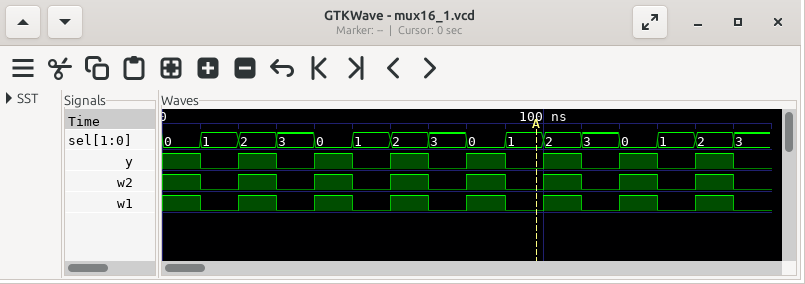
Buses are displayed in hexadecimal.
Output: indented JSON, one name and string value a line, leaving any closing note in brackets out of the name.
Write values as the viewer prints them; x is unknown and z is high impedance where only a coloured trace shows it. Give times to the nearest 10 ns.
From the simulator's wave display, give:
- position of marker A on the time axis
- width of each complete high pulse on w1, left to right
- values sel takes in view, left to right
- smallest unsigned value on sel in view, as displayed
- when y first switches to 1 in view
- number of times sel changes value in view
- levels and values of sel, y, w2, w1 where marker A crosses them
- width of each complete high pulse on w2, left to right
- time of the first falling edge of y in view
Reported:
{
  "position of marker A on the time axis": "100 ns",
  "width of each complete high pulse on w1, left to right": "10 ns, 10 ns, 10 ns, 10 ns, 10 ns, 10 ns, 10 ns",
  "values sel takes in view, left to right": "0, 1, 2, 3, 0, 1, 2, 3, 0, 1, 2, 3, 0, 1, 2, 3",
  "smallest unsigned value on sel in view, as displayed": "0",
  "when y first switches to 1 in view": "20 ns",
  "number of times sel changes value in view": "15",
  "levels and values of sel, y, w2, w1 where marker A crosses them": "sel=1, y=0, w2=0, w1=0",
  "width of each complete high pulse on w2, left to right": "10 ns, 10 ns, 10 ns, 10 ns, 10 ns, 10 ns, 10 ns",
  "time of the first falling edge of y in view": "10 ns"
}
